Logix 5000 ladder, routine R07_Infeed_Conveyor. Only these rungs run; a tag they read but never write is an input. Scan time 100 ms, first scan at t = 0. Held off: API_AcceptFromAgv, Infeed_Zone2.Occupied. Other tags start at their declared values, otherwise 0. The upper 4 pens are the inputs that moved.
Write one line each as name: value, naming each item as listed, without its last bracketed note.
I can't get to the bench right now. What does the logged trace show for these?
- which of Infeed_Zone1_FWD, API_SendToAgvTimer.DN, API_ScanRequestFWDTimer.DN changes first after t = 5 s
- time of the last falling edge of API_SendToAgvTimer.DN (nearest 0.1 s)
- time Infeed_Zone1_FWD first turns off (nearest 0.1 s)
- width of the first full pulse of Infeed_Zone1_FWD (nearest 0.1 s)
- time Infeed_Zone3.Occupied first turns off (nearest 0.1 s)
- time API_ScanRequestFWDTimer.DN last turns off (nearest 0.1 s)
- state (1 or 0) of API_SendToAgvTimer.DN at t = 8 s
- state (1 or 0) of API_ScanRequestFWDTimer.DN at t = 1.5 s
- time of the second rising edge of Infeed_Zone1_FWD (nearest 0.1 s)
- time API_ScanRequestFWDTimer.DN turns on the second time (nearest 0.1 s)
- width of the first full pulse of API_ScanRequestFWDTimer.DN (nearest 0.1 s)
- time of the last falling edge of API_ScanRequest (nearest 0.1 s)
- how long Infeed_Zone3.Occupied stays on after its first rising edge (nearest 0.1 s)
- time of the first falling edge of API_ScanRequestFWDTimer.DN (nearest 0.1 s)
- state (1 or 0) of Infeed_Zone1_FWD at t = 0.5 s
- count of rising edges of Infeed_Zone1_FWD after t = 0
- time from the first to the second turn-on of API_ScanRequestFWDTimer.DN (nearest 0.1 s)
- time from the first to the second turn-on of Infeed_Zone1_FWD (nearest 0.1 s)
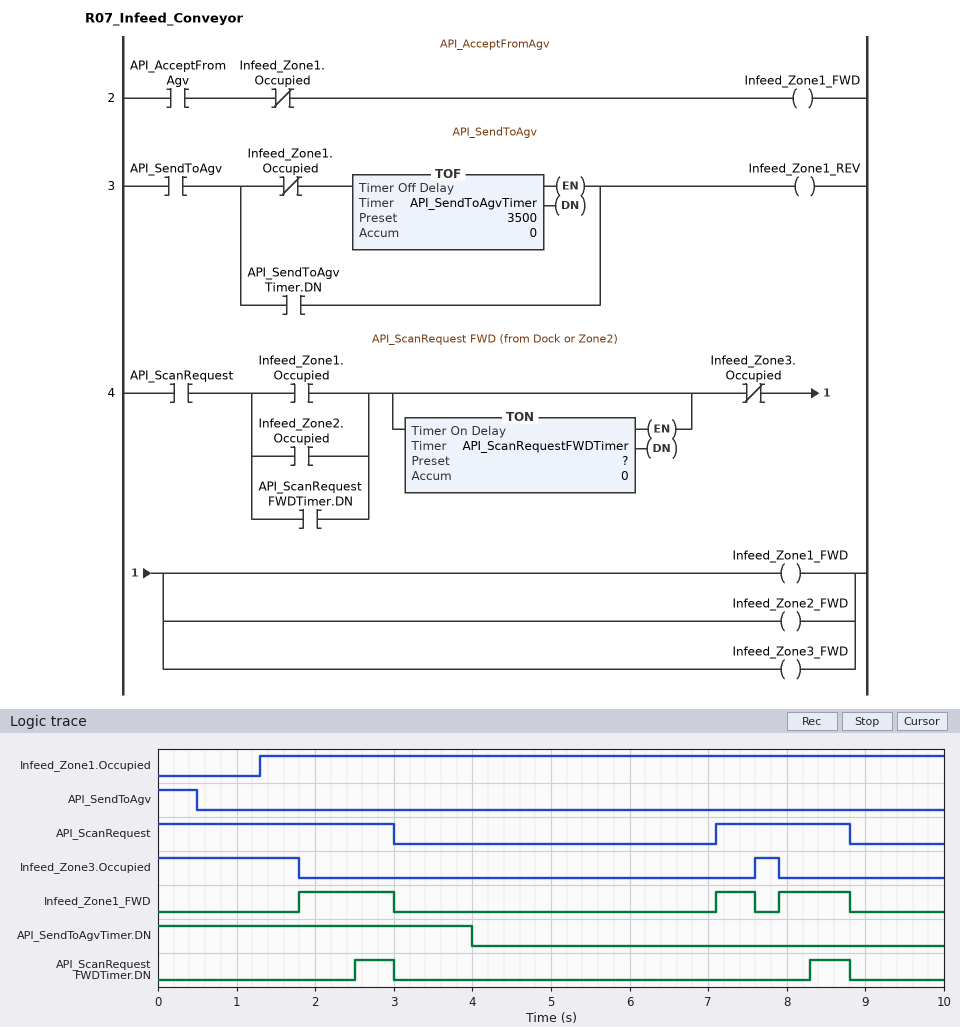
which of Infeed_Zone1_FWD, API_SendToAgvTimer.DN, API_ScanRequestFWDTimer.DN changes first after t = 5 s: Infeed_Zone1_FWD
time of the last falling edge of API_SendToAgvTimer.DN: 4.0 s
time Infeed_Zone1_FWD first turns off: 3.0 s
width of the first full pulse of Infeed_Zone1_FWD: 1.2 s
time Infeed_Zone3.Occupied first turns off: 1.8 s
time API_ScanRequestFWDTimer.DN last turns off: 8.8 s
state (1 or 0) of API_SendToAgvTimer.DN at t = 8 s: 0
state (1 or 0) of API_ScanRequestFWDTimer.DN at t = 1.5 s: 0
time of the second rising edge of Infeed_Zone1_FWD: 7.1 s
time API_ScanRequestFWDTimer.DN turns on the second time: 8.3 s
width of the first full pulse of API_ScanRequestFWDTimer.DN: 0.5 s
time of the last falling edge of API_ScanRequest: 8.8 s
how long Infeed_Zone3.Occupied stays on after its first rising edge: 0.3 s
time of the first falling edge of API_ScanRequestFWDTimer.DN: 3.0 s
state (1 or 0) of Infeed_Zone1_FWD at t = 0.5 s: 0
count of rising edges of Infeed_Zone1_FWD after t = 0: 3
time from the first to the second turn-on of API_ScanRequestFWDTimer.DN: 5.8 s
time from the first to the second turn-on of Infeed_Zone1_FWD: 5.3 s
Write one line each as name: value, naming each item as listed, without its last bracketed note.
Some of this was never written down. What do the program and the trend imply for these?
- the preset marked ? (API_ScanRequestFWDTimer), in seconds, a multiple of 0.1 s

the preset marked ? (API_ScanRequestFWDTimer), in seconds, a multiple of 0.1 s: 1.2 s
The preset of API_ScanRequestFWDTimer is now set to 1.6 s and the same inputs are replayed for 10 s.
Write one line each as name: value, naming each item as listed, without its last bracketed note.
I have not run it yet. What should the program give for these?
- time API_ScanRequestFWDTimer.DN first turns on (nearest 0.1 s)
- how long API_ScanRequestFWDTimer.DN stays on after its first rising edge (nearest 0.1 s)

time API_ScanRequestFWDTimer.DN first turns on: 2.9 s
how long API_ScanRequestFWDTimer.DN stays on after its first rising edge: 0.1 s
